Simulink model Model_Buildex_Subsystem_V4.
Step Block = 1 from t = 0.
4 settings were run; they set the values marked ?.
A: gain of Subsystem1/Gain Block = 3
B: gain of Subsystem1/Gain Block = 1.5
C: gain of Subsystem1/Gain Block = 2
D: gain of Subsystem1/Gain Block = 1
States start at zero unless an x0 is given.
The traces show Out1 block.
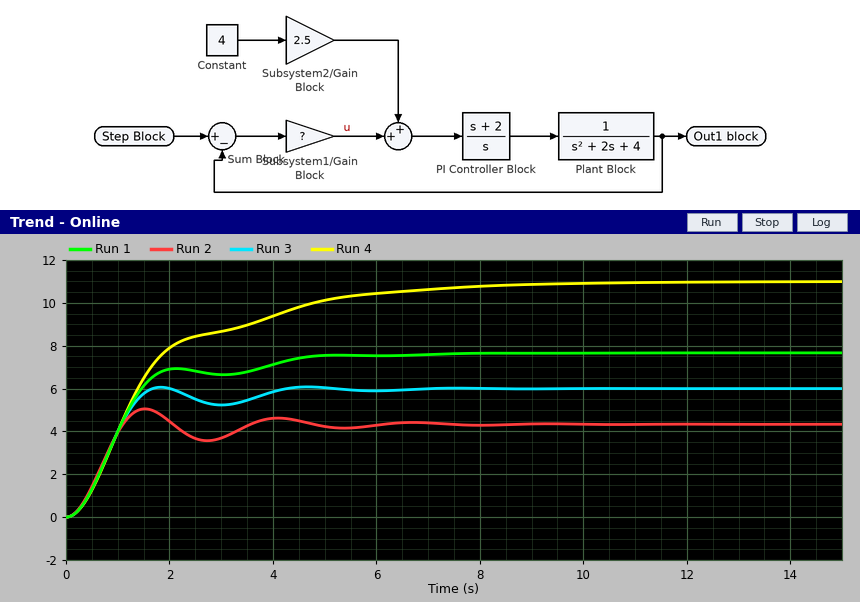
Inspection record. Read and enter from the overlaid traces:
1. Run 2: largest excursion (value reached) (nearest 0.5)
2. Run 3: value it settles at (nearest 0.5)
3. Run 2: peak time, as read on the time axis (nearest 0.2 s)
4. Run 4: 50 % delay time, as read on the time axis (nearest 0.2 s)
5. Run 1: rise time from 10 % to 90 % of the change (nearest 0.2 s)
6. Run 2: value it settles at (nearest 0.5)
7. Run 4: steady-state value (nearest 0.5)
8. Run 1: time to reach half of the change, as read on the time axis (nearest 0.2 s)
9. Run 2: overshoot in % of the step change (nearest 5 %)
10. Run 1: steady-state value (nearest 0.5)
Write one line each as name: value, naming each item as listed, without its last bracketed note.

Run 2: largest excursion (value reached): 5.0
Run 3: value it settles at: 6.0
Run 2: peak time, as read on the time axis: 1.6 s
Run 4: 50 % delay time, as read on the time axis: 1.2 s
Run 1: rise time from 10 % to 90 % of the change: 1.6 s
Run 2: value it settles at: 4.5
Run 4: steady-state value: 11.0
Run 1: time to reach half of the change, as read on the time axis: 1.0 s
Run 2: overshoot in % of the step change: 15 %
Run 1: steady-state value: 7.5
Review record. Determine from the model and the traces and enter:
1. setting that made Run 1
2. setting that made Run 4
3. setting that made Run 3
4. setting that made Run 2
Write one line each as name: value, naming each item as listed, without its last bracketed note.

setting that made Run 1: B
setting that made Run 4: D
setting that made Run 3: C
setting that made Run 2: A
